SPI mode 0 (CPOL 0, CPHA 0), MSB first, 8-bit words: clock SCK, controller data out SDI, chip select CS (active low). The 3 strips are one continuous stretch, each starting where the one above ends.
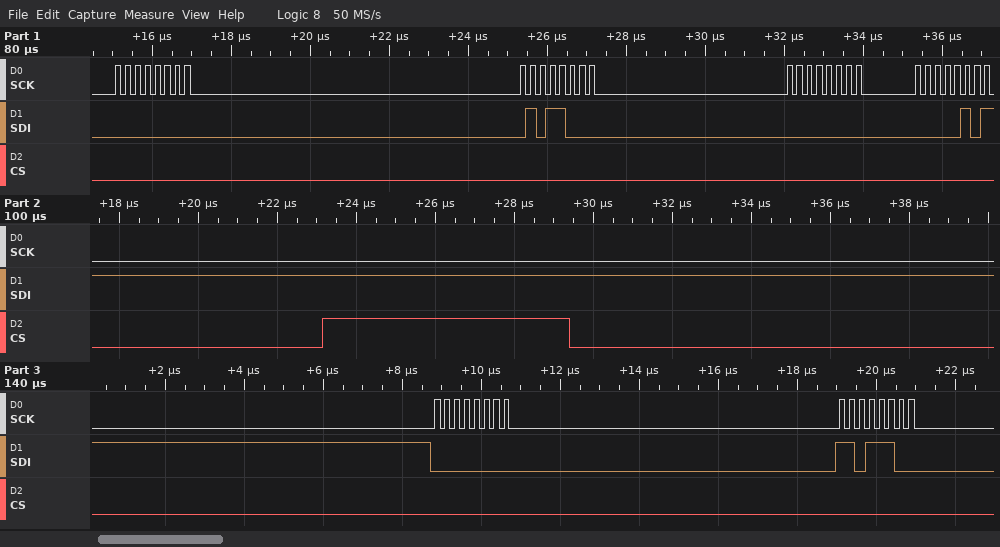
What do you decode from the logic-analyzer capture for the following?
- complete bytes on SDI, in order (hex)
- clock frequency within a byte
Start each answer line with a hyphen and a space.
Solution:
- 00 58 00 05 00 DC
- 4 MHz
